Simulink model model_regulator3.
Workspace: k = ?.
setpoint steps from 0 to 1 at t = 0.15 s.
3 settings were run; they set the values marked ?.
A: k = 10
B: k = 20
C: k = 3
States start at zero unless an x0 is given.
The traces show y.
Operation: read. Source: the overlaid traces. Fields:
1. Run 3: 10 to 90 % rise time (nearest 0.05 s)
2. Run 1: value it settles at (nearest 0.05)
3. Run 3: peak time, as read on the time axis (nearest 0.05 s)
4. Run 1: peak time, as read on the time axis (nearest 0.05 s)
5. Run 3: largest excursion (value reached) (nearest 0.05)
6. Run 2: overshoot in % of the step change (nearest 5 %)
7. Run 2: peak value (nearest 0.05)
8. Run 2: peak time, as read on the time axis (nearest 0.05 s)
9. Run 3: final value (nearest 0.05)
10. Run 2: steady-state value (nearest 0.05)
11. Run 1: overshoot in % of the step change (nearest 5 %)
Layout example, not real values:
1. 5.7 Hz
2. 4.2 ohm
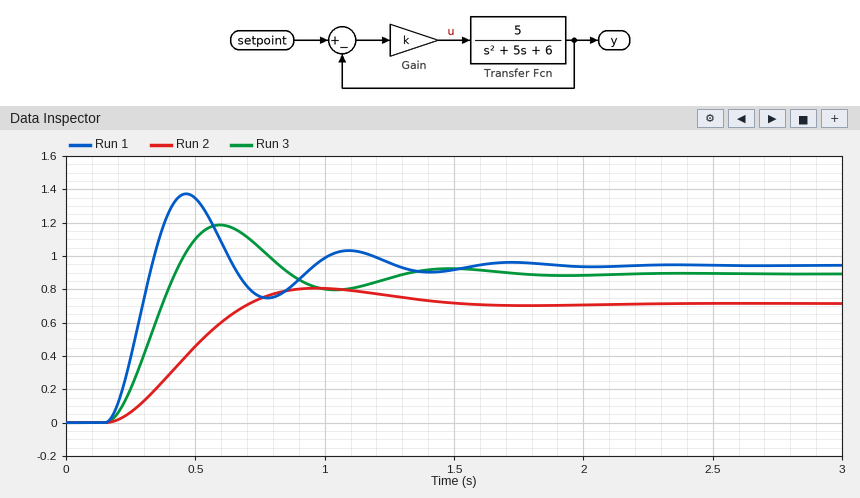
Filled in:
1. 0.20 s
2. 0.95
3. 0.60 s
4. 0.45 s
5. 1.20
6. 15 %
7. 0.80
8. 0.95 s
9. 0.90
10. 0.70
11. 45 %
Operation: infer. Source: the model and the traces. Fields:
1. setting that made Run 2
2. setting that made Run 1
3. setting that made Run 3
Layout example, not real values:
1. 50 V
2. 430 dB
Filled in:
1. C
2. B
3. A
